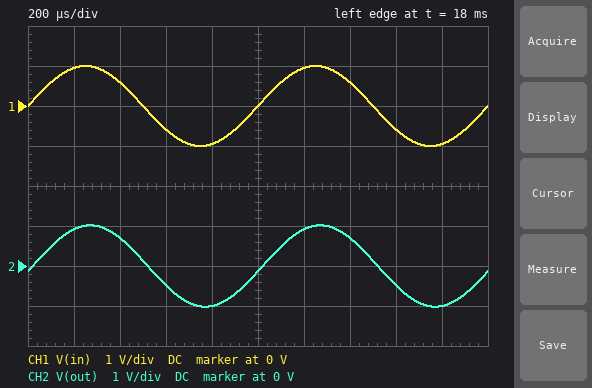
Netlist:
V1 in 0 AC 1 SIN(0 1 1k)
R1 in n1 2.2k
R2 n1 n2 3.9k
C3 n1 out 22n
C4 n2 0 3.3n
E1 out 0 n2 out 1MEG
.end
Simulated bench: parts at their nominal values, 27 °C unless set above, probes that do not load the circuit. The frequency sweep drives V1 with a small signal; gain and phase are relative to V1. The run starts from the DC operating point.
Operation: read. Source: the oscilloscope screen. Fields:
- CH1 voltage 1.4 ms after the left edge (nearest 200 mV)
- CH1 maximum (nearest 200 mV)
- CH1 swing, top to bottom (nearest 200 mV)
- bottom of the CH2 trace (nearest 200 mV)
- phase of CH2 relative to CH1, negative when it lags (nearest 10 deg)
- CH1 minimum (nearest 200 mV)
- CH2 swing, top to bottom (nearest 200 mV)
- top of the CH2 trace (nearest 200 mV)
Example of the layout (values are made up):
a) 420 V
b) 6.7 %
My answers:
a) 600 mV
b) 1.0 V
c) 2.0 V
d) -1.0 V
e) -10 deg
f) -1.0 V
g) 2.0 V
h) 1.0 V
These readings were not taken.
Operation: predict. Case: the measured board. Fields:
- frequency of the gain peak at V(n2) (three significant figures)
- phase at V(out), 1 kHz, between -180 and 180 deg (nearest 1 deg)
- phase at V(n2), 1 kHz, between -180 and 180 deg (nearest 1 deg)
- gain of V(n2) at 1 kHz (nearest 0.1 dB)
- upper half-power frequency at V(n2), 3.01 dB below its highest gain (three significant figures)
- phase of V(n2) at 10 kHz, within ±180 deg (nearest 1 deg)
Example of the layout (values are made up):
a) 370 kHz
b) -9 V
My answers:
a) 5.24 kHz
b) -7 deg
c) -7 deg
d) 0.1 dB
e) 7.58 kHz
f) -139 deg
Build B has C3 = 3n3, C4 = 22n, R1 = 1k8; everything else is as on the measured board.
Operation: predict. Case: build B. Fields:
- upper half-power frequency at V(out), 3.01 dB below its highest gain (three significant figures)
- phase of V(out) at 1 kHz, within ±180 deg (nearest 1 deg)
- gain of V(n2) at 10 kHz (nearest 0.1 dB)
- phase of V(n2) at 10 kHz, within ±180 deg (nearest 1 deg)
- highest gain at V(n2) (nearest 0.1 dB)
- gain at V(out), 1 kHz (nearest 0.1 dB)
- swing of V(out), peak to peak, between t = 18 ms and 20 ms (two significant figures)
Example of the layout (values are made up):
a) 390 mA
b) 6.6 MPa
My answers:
a) 1.31 kHz
b) -39 deg
c) -18.0 dB
d) -97 deg
e) 0 dB
f) -2.0 dB
g) 1.6 V
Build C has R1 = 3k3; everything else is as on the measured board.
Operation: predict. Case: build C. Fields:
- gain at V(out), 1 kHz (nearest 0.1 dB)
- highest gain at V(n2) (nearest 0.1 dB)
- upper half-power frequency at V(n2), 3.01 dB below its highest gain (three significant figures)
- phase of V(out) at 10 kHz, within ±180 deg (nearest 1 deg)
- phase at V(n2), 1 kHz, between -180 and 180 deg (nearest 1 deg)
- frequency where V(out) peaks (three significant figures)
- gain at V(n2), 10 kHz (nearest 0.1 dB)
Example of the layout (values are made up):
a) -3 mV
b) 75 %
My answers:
a) 0.2 dB
b) 2.9 dB
c) 6.19 kHz
d) -151 deg
e) -9 deg
f) 4.35 kHz
g) -9.8 dB
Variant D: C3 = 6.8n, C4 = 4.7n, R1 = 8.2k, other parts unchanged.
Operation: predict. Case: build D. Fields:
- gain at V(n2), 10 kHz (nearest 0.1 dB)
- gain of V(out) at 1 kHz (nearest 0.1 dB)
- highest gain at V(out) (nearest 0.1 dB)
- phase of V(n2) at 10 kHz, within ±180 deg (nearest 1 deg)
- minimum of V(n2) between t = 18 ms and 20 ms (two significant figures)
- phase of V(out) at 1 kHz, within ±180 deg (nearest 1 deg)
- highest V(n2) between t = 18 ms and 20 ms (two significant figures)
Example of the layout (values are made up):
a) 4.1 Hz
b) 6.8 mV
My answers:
a) -13.4 dB
b) -0.2 dB
c) 0 dB
d) -130 deg
e) -980 mV
f) -20 deg
g) 980 mV
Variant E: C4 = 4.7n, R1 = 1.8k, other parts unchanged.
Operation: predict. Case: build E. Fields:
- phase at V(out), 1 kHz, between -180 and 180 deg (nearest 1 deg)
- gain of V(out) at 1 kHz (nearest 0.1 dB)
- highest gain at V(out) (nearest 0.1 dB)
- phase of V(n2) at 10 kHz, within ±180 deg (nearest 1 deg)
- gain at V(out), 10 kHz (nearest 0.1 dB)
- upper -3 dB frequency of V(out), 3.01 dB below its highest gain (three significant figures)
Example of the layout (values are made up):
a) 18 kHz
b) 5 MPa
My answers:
a) -10 deg
b) 0.1 dB
c) 1.3 dB
d) -138 deg
e) -8.0 dB
f) 6.91 kHz
